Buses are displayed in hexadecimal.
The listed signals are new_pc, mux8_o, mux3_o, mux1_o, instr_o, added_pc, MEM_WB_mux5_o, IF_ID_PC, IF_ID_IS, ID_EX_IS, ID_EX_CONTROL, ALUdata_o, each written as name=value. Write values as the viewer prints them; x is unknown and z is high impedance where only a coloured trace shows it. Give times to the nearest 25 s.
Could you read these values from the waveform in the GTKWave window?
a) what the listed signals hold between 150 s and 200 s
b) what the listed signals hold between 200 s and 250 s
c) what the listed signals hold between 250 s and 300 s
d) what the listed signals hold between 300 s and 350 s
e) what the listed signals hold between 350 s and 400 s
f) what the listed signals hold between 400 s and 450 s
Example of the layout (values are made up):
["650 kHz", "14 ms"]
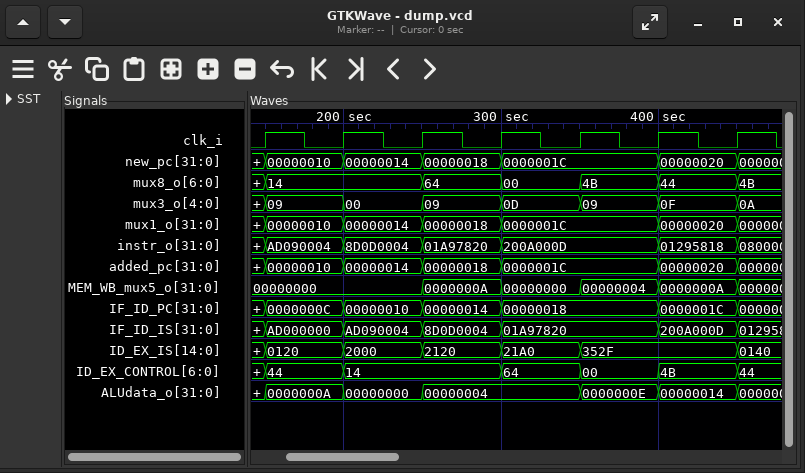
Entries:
["new_pc=00000010, mux8_o=14, mux3_o=09, mux1_o=00000010, instr_o=AD090004, added_pc=00000010, MEM_WB_mux5_o=00000000, IF_ID_PC=0000000C, IF_ID_IS=AD000000, ID_EX_IS=0120, ID_EX_CONTROL=44, ALUdata_o=0000000A", "new_pc=00000014, mux8_o=14, mux3_o=00, mux1_o=00000014, instr_o=8D0D0004, added_pc=00000014, MEM_WB_mux5_o=00000000, IF_ID_PC=00000010, IF_ID_IS=AD090004, ID_EX_IS=2000, ID_EX_CONTROL=14, ALUdata_o=00000000", "new_pc=00000018, mux8_o=64, mux3_o=09, mux1_o=00000018, instr_o=01A97820, added_pc=00000018, MEM_WB_mux5_o=0000000A, IF_ID_PC=00000014, IF_ID_IS=8D0D0004, ID_EX_IS=2120, ID_EX_CONTROL=14, ALUdata_o=00000004", "new_pc=0000001C, mux8_o=00, mux3_o=0D, mux1_o=0000001C, instr_o=200A000D, added_pc=0000001C, MEM_WB_mux5_o=00000000, IF_ID_PC=00000018, IF_ID_IS=01A97820, ID_EX_IS=21A0, ID_EX_CONTROL=64, ALUdata_o=00000004", "new_pc=0000001C, mux8_o=4B, mux3_o=09, mux1_o=0000001C, instr_o=200A000D, added_pc=0000001C, MEM_WB_mux5_o=00000004, IF_ID_PC=00000018, IF_ID_IS=01A97820, ID_EX_IS=352F, ID_EX_CONTROL=00, ALUdata_o=0000000E", "new_pc=00000020, mux8_o=44, mux3_o=0F, mux1_o=00000020, instr_o=01295818, added_pc=00000020, MEM_WB_mux5_o=0000000A, IF_ID_PC=0000001C, IF_ID_IS=200A000D, ID_EX_IS=352F, ID_EX_CONTROL=4B, ALUdata_o=00000014"]
